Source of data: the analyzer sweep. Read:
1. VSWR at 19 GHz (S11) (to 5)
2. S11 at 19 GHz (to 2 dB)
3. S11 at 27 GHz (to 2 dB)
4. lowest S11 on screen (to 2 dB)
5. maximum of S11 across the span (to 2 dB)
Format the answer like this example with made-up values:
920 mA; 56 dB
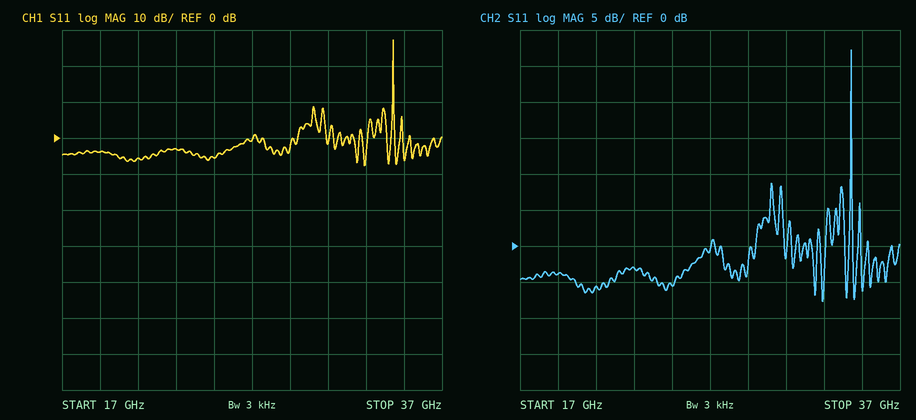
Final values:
5; -4 dB; 0 dB; -8 dB; 28 dB
